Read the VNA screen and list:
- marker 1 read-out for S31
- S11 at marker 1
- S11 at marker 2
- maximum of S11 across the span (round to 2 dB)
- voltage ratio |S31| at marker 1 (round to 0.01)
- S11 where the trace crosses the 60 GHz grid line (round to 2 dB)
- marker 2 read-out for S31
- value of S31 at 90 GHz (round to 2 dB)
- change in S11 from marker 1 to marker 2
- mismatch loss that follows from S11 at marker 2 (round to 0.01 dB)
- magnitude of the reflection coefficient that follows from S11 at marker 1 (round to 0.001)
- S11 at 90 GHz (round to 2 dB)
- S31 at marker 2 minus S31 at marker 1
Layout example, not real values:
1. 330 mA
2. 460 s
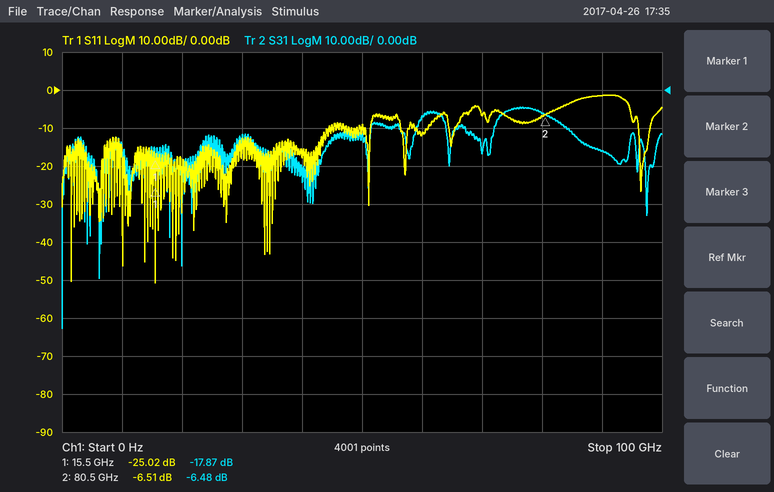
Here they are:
1. -17.87 dB
2. -25.02 dB
3. -6.51 dB
4. -2 dB
5. 0.13
6. -12 dB
7. -6.48 dB
8. -16 dB
9. 18.51 dB
10. 1.10 dB
11. 0.056
12. -2 dB
13. 11.39 dB
